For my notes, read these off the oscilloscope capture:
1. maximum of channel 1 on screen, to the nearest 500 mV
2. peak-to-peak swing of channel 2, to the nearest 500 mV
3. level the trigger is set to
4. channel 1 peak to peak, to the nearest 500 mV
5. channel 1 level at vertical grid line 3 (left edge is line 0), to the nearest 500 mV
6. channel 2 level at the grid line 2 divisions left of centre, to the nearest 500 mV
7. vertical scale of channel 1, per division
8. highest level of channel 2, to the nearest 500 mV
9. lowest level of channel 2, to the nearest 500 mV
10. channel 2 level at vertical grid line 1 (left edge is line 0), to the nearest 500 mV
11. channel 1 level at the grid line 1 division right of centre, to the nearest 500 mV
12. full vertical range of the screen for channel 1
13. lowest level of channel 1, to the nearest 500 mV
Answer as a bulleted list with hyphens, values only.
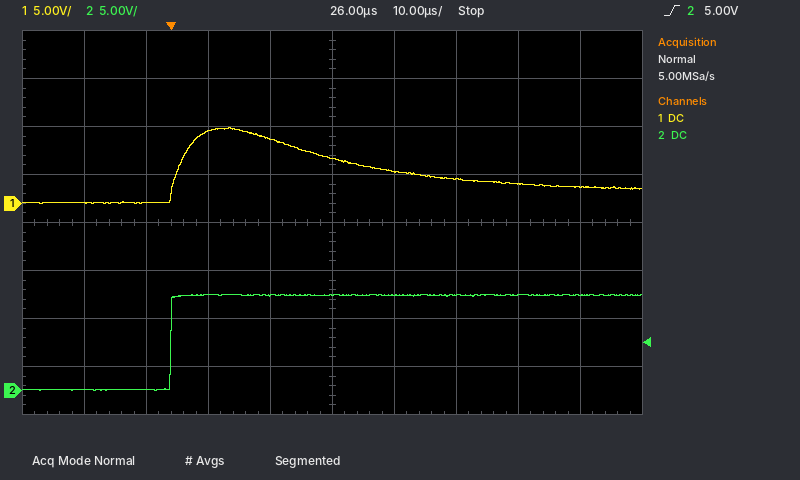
- 8.0 V
- 10.0 V
- 5.00 V
- 8.0 V
- 7.5 V
- 10.0 V
- 5 V
- 10.0 V
- 0.0 V
- 0.0 V
- 3.5 V
- 40 V
- 0.0 V
